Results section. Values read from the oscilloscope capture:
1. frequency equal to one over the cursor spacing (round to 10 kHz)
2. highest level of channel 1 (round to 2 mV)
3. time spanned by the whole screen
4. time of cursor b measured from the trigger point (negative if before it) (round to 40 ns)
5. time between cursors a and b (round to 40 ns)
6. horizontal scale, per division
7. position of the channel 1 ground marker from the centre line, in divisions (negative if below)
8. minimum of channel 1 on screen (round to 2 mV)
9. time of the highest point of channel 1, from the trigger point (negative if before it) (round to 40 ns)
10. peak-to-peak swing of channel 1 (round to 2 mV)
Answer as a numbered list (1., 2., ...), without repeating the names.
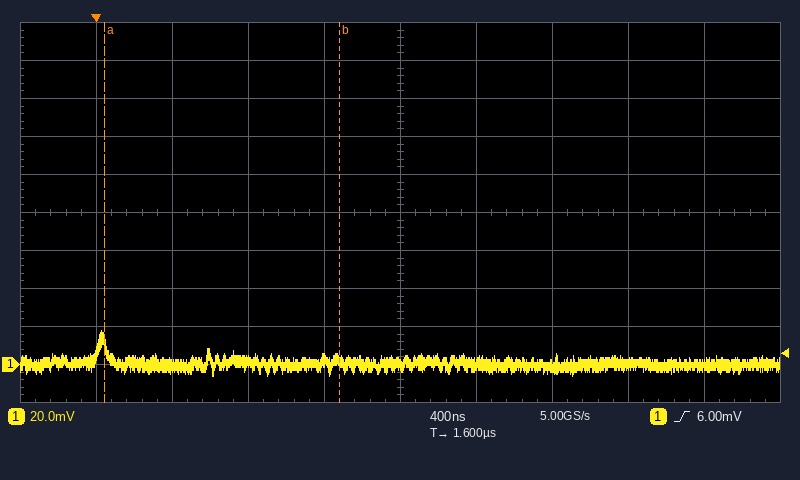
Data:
1. 810 kHz
2. 18 mV
3. 4 µs
4. +1.28 µs
5. 1.24 µs
6. 400 ns
7. -4.0 div
8. -6 mV
9. +40 ns
10. 24 mV
